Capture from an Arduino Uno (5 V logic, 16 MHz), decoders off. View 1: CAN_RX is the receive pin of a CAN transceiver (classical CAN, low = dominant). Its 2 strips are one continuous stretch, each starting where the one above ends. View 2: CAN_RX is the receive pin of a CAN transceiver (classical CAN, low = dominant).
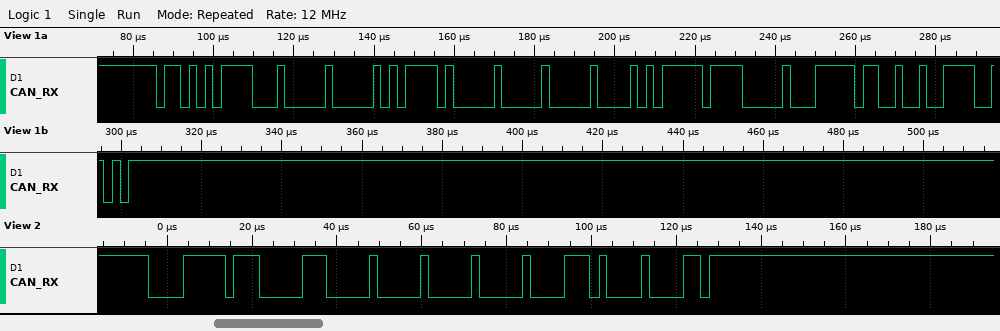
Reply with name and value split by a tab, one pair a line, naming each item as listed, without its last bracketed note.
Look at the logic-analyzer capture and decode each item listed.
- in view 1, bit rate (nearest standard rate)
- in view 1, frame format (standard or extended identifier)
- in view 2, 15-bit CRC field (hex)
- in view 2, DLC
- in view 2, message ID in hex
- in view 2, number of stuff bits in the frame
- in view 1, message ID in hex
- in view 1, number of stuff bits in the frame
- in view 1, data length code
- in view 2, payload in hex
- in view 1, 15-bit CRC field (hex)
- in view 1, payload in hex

in view 1, bit rate	500 kbit/s
in view 1, frame format	standard
in view 2, 15-bit CRC field	0x7421
in view 2, DLC	3
in view 2, message ID in hex	0x0FF
in view 2, number of stuff bits in the frame	6
in view 1, message ID in hex	0x6AF
in view 1, number of stuff bits in the frame	8
in view 1, data length code	8
in view 2, payload in hex	00 00 00
in view 1, 15-bit CRC field	0x24F2
in view 1, payload in hex	00 BD 00 00 15 FF 00 FE
